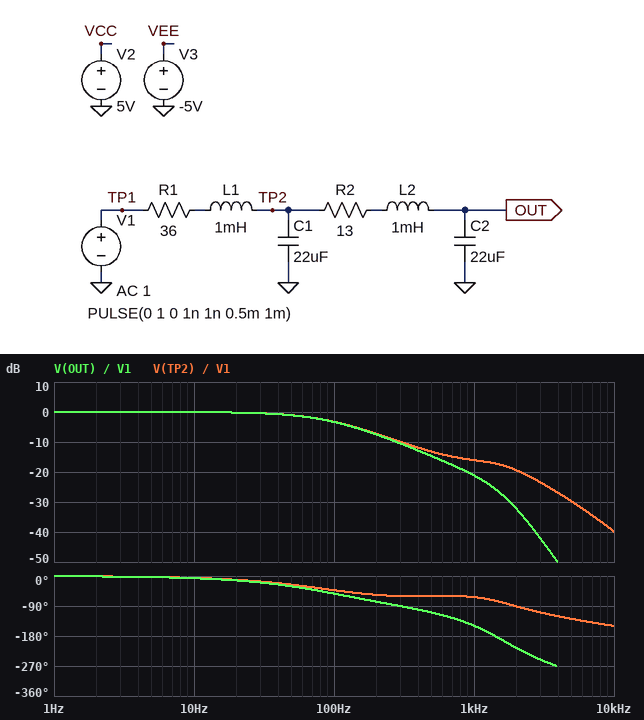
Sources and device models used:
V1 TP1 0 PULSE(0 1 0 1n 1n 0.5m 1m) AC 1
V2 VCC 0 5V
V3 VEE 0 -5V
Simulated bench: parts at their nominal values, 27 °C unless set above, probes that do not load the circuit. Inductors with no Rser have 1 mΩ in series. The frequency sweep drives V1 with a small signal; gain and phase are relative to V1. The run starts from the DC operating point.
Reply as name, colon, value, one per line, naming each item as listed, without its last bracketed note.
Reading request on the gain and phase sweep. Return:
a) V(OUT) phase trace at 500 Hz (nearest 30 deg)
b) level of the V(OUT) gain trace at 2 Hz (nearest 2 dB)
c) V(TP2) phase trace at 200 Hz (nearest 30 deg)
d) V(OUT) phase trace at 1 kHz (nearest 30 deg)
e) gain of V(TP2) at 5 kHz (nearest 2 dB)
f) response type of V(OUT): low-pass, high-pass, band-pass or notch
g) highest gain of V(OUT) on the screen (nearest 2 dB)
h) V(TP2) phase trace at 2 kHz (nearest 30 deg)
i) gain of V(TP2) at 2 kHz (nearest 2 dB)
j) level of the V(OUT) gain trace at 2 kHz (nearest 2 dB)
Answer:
V(OUT) phase trace at 500 Hz: -120 deg
level of the V(OUT) gain trace at 2 Hz: 0 dB
V(TP2) phase trace at 200 Hz: -60 deg
V(OUT) phase trace at 1 kHz: -150 deg
gain of V(TP2) at 5 kHz: -30 dB
response type of V(OUT): low-pass, high-pass, band-pass or notch: low-pass
highest gain of V(OUT) on the screen: 0 dB
V(TP2) phase trace at 2 kHz: -90 deg
gain of V(TP2) at 2 kHz: -20 dB
level of the V(OUT) gain trace at 2 kHz: -32 dB
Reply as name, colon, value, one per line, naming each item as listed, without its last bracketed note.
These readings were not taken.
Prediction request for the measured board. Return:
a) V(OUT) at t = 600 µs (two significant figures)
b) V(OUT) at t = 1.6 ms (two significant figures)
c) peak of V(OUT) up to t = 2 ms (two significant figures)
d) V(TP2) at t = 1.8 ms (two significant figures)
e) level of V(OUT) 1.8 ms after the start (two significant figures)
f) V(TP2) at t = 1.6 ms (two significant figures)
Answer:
V(OUT) at t = 600 µs: 220 mV
V(OUT) at t = 1.6 ms: 370 mV
peak of V(OUT) up to t = 2 ms: 380 mV
V(TP2) at t = 1.8 ms: 300 mV
level of V(OUT) 1.8 ms after the start: 370 mV
V(TP2) at t = 1.6 ms: 390 mV
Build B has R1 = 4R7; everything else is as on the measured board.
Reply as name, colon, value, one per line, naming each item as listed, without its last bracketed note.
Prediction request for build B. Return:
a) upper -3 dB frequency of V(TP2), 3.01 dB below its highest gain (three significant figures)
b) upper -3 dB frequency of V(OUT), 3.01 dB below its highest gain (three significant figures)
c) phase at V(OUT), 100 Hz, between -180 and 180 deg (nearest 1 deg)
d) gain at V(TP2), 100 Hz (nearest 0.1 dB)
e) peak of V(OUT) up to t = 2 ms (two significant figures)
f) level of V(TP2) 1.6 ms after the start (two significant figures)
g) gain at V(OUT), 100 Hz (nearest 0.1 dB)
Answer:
upper -3 dB frequency of V(TP2), 3.01 dB below its highest gain: 1.35 kHz
upper -3 dB frequency of V(OUT), 3.01 dB below its highest gain: 594 Hz
phase at V(OUT), 100 Hz, between -180 and 180 deg: -18 deg
gain at V(TP2), 100 Hz: 0 dB
peak of V(OUT) up to t = 2 ms: 790 mV
level of V(TP2) 1.6 ms after the start: 800 mV
gain at V(OUT), 100 Hz: -0.1 dB
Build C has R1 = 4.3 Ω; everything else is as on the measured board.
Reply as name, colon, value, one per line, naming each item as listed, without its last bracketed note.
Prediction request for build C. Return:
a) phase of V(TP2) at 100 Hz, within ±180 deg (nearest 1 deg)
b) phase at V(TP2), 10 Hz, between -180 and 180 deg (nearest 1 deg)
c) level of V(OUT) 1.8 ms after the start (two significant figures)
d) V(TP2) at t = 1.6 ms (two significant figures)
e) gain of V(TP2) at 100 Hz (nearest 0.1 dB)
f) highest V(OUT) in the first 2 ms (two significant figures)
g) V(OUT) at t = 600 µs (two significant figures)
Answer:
phase of V(TP2) at 100 Hz, within ±180 deg: -7 deg
phase at V(TP2), 10 Hz, between -180 and 180 deg: -1 deg
level of V(OUT) 1.8 ms after the start: 720 mV
V(TP2) at t = 1.6 ms: 820 mV
gain of V(TP2) at 100 Hz: 0 dB
highest V(OUT) in the first 2 ms: 800 mV
V(OUT) at t = 600 µs: 750 mV
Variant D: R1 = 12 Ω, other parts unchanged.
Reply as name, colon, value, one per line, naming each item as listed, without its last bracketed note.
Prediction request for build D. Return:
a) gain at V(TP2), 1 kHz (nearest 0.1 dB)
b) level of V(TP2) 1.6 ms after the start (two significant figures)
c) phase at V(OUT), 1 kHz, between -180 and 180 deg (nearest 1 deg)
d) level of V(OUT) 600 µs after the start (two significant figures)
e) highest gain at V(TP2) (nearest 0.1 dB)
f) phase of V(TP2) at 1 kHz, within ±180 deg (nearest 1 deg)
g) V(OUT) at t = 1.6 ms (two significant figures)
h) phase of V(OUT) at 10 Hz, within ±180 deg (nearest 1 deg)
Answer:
gain at V(TP2), 1 kHz: -7.7 dB
level of V(TP2) 1.6 ms after the start: 620 mV
phase at V(OUT), 1 kHz, between -180 and 180 deg: -151 deg
level of V(OUT) 600 µs after the start: 470 mV
highest gain at V(TP2): 0 dB
phase of V(TP2) at 1 kHz, within ±180 deg: -65 deg
V(OUT) at t = 1.6 ms: 600 mV
phase of V(OUT) at 10 Hz, within ±180 deg: -3 deg
